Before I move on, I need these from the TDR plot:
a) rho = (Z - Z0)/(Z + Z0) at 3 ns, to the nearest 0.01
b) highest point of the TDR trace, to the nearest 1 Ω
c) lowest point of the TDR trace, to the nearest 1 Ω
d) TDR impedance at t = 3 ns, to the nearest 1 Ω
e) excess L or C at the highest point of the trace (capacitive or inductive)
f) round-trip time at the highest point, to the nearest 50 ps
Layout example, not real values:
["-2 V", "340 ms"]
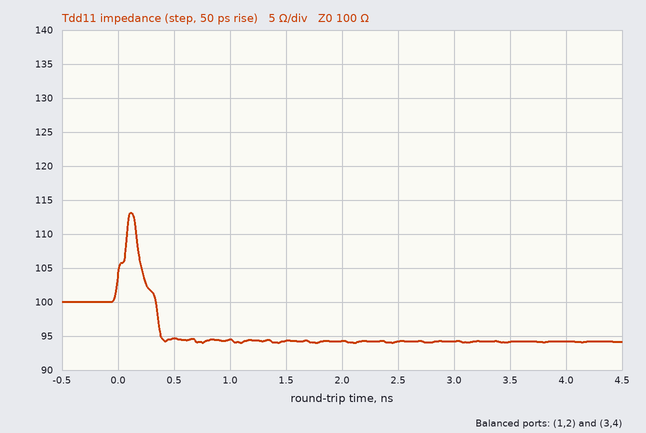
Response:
["-0.03", "113 Ω", "94 Ω", "94 Ω", "inductive", "100 ps"]
